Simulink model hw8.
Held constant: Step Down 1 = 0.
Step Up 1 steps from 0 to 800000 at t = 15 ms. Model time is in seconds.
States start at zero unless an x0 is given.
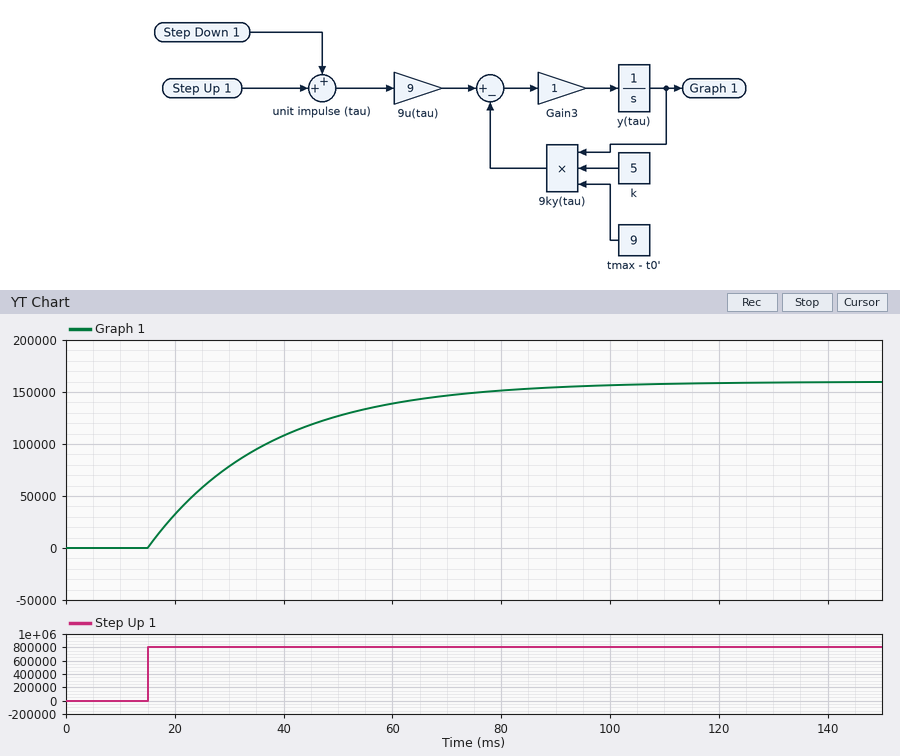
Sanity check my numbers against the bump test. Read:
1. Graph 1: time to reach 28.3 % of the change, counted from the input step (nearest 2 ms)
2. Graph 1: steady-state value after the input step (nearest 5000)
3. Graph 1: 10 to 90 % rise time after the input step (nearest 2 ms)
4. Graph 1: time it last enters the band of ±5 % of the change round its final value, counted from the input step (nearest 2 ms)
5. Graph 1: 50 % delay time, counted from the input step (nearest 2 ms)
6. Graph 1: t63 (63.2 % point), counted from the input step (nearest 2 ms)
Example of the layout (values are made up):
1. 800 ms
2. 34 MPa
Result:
1. 8 ms
2. 160000
3. 48 ms
4. 66 ms
5. 16 ms
6. 22 ms
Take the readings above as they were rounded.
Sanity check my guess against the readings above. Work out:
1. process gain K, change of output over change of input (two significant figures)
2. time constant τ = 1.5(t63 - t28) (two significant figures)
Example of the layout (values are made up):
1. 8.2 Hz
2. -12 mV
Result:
1. 0.20
2. 21 ms
